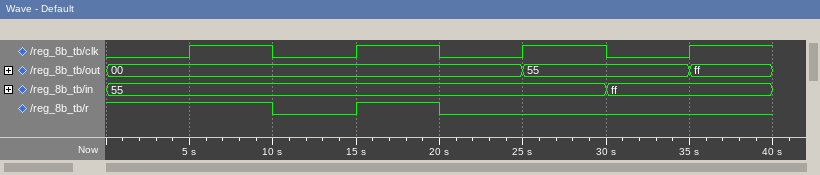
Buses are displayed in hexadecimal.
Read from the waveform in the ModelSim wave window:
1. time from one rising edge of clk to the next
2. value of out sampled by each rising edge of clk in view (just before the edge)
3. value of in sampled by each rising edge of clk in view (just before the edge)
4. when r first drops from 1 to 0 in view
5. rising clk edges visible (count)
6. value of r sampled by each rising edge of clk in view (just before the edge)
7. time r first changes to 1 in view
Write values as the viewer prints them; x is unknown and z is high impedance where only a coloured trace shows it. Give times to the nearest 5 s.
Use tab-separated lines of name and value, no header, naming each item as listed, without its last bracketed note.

time from one rising edge of clk to the next	10 s
value of out sampled by each rising edge of clk in view	00, 00, 00, 55
value of in sampled by each rising edge of clk in view	55, 55, 55, ff
when r first drops from 1 to 0 in view	10 s
rising clk edges visible	4
value of r sampled by each rising edge of clk in view	1 0 0 0
time r first changes to 1 in view	15 s
